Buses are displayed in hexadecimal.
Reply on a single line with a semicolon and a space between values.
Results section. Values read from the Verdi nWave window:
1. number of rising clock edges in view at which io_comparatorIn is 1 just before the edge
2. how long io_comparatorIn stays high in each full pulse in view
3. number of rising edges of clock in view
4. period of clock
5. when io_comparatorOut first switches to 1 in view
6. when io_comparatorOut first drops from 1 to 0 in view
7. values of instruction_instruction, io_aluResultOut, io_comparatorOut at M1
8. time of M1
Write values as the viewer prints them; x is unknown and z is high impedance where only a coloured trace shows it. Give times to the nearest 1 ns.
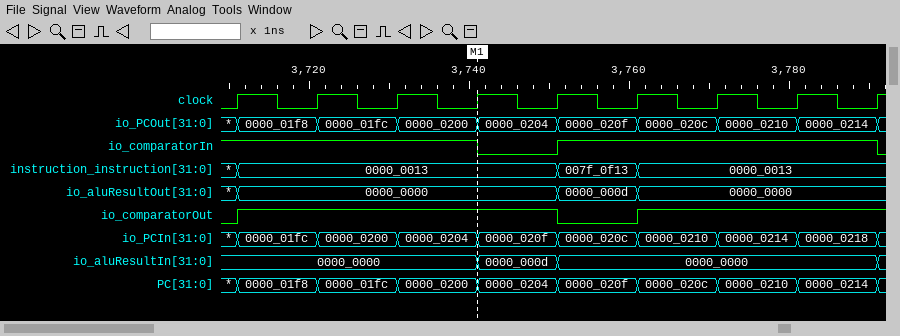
8; 40 ns; 9; 10 ns; 3711 ns; 3751 ns; instruction_instruction=0000_0013, io_aluResultOut=0000_0000, io_comparatorOut=1; 3741 ns
